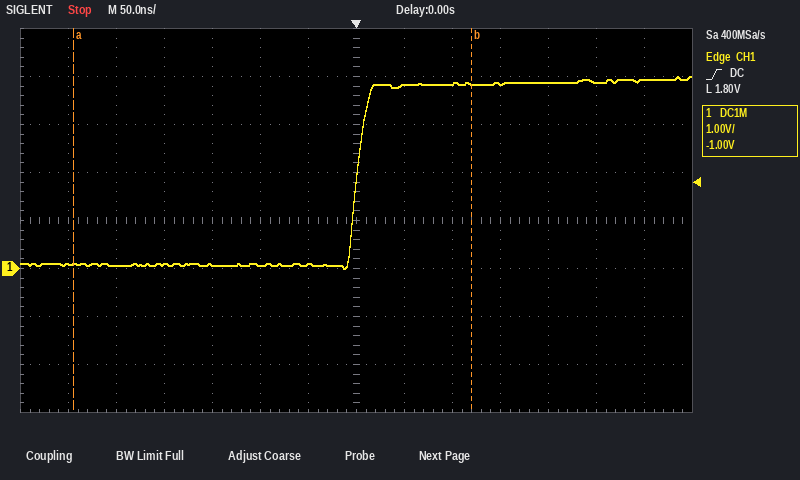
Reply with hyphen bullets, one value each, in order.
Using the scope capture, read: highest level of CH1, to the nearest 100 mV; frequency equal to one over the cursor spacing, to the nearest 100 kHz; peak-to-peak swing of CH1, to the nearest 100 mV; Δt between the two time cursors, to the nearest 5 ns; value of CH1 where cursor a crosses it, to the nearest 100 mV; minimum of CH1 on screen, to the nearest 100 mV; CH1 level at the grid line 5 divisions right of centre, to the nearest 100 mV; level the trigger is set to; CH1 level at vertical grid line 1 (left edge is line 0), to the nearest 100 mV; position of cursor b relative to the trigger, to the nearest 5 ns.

- 4.0 V
- 2.4 MHz
- 4.0 V
- 415 ns
- 100 mV
- 0.0 V
- 3.9 V
- 1.80 V
- 100 mV
- +120 ns
